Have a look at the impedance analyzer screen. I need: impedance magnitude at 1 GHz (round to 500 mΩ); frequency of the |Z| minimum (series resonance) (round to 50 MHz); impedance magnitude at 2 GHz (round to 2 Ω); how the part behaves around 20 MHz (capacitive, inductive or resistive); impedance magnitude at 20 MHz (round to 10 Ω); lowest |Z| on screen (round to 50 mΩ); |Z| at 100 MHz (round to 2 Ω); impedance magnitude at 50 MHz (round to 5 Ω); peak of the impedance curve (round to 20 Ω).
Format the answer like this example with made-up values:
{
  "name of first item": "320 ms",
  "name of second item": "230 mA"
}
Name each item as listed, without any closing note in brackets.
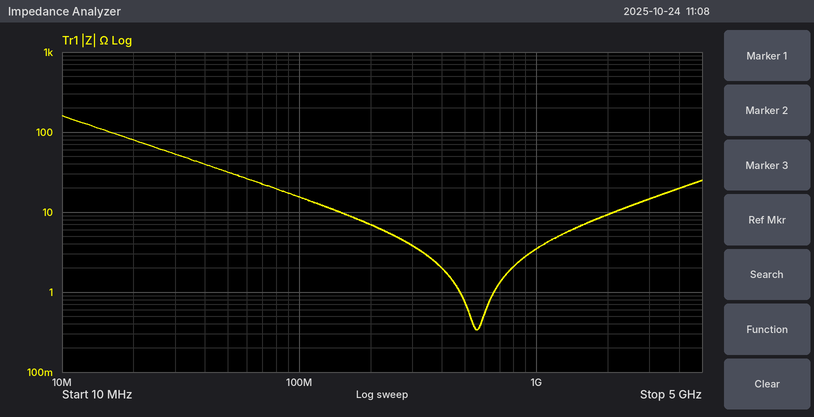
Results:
{
  "impedance magnitude at 1 GHz": "3.5 Ω",
  "frequency of the |Z| minimum (series resonance)": "550 MHz",
  "impedance magnitude at 2 GHz": "10 Ω",
  "how the part behaves around 20 MHz": "capacitive",
  "impedance magnitude at 20 MHz": "80 Ω",
  "lowest |Z| on screen": "350 mΩ",
  "|Z| at 100 MHz": "16 Ω",
  "impedance magnitude at 50 MHz": "30 Ω",
  "peak of the impedance curve": "160 Ω"
}
